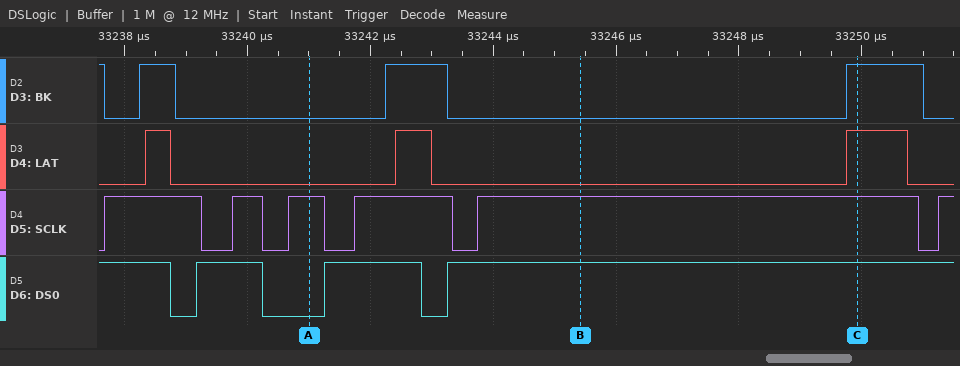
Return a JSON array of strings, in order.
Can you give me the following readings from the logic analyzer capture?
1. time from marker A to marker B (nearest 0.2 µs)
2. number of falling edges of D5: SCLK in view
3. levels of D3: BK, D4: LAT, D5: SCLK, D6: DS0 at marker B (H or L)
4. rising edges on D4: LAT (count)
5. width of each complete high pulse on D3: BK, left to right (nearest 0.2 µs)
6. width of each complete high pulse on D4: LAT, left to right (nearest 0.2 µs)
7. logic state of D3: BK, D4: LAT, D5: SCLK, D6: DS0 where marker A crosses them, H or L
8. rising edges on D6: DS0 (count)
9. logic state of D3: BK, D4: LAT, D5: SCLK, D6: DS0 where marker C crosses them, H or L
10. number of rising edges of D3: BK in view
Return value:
["4.4 µs", "5", "D3: BK=L, D4: LAT=L, D5: SCLK=H, D6: DS0=H", "3", "0.6 µs, 1 µs, 1.2 µs", "0.4 µs, 0.6 µs, 1 µs", "D3: BK=L, D4: LAT=L, D5: SCLK=H, D6: DS0=L", "3", "D3: BK=H, D4: LAT=H, D5: SCLK=H, D6: DS0=H", "3"]
